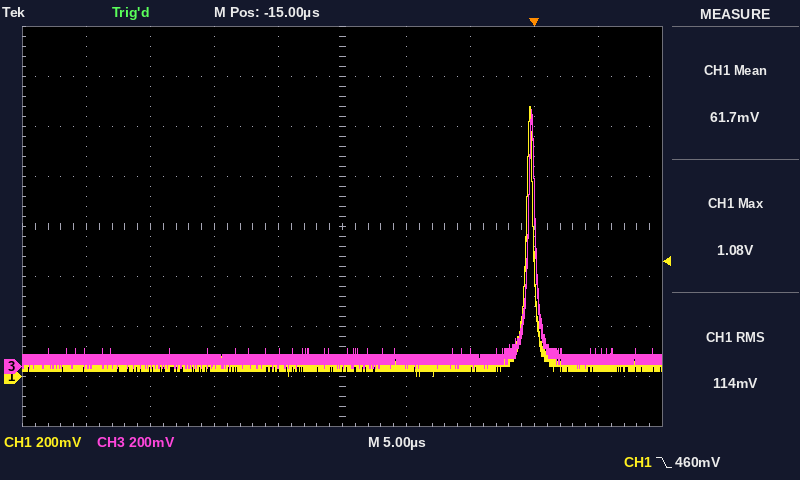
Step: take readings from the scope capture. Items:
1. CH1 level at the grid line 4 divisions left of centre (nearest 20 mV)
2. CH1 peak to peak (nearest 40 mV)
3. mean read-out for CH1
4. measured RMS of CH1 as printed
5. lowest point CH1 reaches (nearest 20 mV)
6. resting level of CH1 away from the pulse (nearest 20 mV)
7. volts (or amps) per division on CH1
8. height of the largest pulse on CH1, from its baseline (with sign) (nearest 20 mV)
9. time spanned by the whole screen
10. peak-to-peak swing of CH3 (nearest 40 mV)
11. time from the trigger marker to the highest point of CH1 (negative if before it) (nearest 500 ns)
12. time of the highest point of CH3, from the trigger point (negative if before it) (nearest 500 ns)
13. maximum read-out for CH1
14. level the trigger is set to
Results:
40 mV
1.08 V
61.7 mV
114 mV
0 mV
40 mV
200 mV
+1.04 V
50 µs
1.04 V
-500 ns
0.0 µs
1.08 V
460 mV
